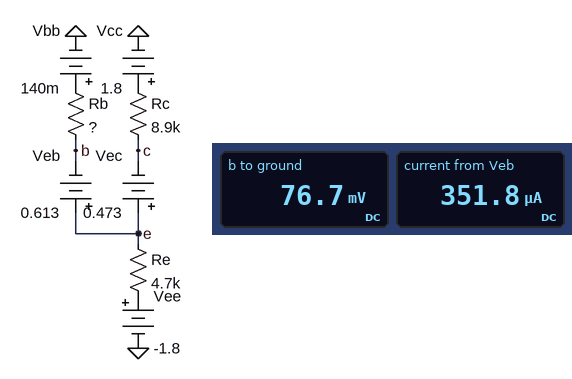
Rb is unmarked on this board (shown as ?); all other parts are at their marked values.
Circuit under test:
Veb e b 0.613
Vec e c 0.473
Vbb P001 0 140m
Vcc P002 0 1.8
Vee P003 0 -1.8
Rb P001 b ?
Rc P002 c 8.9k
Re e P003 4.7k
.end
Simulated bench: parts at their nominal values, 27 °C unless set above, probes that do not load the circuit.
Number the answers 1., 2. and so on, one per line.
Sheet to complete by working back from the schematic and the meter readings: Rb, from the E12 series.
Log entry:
1. 180 Ω
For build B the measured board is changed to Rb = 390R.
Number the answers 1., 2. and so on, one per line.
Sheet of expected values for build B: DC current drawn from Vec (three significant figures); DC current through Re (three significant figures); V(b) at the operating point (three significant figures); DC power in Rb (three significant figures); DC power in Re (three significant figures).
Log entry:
1. 185 µA
2. 516 µA
3. 11.1 mV
4. 42.6 µW
5. 1.25 mW
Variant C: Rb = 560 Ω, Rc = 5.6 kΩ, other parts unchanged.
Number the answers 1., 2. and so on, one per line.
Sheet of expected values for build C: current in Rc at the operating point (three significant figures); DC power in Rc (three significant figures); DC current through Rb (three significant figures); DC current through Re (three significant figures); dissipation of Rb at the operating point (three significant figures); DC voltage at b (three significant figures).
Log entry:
1. 294 µA
2. 483 µW
3. 223 µA
4. 517 µA
5. 27.8 µW
6. 15.2 mV
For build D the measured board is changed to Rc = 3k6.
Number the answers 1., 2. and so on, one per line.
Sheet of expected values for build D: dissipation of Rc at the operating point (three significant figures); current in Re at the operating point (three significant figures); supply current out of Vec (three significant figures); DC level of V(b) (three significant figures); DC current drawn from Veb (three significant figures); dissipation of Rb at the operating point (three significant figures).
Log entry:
1. 659 µW
2. 539 µA
3. 428 µA
4. 120 mV
5. 111 µA
6. 2.22 µW
